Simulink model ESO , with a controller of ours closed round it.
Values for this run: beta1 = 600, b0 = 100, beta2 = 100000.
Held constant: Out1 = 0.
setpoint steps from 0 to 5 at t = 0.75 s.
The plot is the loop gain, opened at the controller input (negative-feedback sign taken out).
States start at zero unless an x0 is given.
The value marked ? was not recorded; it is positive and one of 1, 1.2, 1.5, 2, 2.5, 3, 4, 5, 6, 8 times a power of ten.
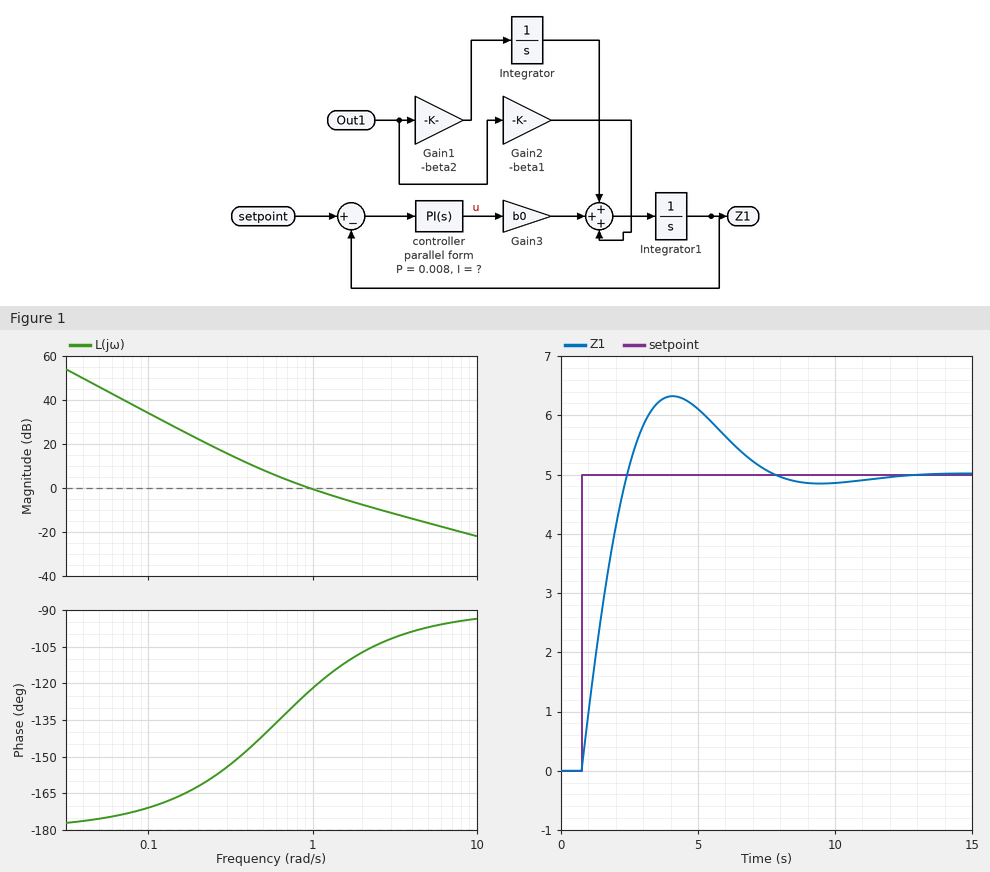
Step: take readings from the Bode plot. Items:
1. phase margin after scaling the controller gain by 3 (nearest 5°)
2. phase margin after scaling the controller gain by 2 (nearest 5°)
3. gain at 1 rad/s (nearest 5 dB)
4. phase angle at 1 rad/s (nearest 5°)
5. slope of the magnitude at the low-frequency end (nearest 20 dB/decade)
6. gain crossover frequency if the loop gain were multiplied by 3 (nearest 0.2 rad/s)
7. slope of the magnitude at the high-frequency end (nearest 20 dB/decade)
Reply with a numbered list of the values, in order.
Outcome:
1. 75°
2. 70°
3. 0 dB
4. -120°
5. -40 dB/decade
6. 2.4 rad/s
7. -20 dB/decade
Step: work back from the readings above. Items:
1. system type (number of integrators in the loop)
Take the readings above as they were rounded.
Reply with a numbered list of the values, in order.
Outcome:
1. 2
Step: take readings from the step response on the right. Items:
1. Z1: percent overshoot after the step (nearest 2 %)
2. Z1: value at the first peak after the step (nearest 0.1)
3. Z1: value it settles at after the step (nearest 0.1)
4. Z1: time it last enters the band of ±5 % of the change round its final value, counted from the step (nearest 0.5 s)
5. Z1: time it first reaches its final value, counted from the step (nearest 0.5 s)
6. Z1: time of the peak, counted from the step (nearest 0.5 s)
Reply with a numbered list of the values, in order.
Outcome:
1. 26 %
2. 6.3
3. 5.0
4. 6.0 s
5. 1.5 s
6. 3.5 s
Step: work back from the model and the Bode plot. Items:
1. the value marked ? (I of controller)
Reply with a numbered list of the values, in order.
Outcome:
1. 0.005
